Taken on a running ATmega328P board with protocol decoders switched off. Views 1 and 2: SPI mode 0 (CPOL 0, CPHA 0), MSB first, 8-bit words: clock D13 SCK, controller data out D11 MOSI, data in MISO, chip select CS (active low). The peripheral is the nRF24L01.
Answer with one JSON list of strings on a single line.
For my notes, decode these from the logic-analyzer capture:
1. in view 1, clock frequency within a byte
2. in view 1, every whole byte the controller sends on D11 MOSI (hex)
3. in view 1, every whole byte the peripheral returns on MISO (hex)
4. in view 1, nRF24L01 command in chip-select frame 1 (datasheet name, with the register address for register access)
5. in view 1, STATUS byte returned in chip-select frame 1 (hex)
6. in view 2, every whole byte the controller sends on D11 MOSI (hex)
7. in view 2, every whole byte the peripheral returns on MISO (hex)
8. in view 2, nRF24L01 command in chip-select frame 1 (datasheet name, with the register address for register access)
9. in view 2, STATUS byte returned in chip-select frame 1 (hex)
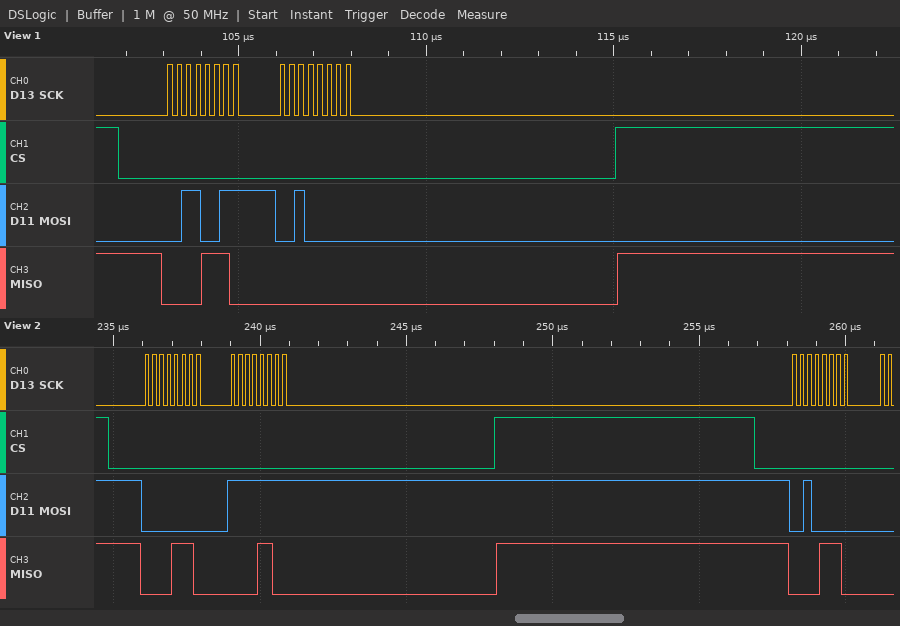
["4 MHz", "0x33 0x20", "0x0E 0x00", "W_REGISTER 0x13", "0x0E", "0x00 0xFF 0x20", "0x0E 0x0C 0x0E", "R_REGISTER 0x00", "0x0E"]
